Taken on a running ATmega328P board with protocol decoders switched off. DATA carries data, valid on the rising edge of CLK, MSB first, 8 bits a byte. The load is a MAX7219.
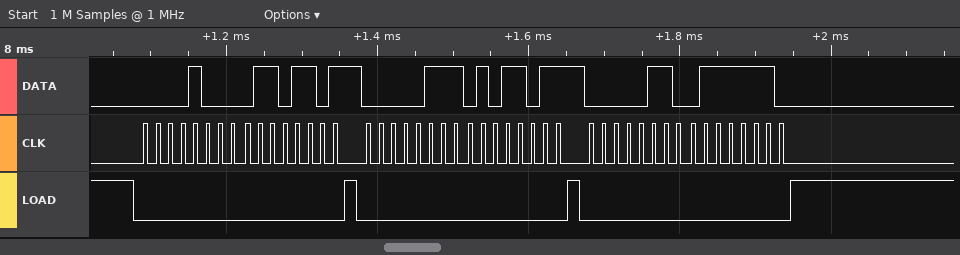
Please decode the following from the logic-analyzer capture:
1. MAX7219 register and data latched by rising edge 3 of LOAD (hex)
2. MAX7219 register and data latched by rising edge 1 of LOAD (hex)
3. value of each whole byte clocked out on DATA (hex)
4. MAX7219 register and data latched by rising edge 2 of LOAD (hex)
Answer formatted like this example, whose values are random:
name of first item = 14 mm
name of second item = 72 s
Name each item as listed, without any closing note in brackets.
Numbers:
MAX7219 register and data latched by rising edge 3 of LOAD = register 0x6, data 0x7E
MAX7219 register and data latched by rising edge 1 of LOAD = register 0x8, data 0x6D
value of each whole byte clocked out on DATA = 0x08 0x6D 0x07 0x5B 0x06 0x7E
MAX7219 register and data latched by rising edge 2 of LOAD = register 0x7, data 0x5B
